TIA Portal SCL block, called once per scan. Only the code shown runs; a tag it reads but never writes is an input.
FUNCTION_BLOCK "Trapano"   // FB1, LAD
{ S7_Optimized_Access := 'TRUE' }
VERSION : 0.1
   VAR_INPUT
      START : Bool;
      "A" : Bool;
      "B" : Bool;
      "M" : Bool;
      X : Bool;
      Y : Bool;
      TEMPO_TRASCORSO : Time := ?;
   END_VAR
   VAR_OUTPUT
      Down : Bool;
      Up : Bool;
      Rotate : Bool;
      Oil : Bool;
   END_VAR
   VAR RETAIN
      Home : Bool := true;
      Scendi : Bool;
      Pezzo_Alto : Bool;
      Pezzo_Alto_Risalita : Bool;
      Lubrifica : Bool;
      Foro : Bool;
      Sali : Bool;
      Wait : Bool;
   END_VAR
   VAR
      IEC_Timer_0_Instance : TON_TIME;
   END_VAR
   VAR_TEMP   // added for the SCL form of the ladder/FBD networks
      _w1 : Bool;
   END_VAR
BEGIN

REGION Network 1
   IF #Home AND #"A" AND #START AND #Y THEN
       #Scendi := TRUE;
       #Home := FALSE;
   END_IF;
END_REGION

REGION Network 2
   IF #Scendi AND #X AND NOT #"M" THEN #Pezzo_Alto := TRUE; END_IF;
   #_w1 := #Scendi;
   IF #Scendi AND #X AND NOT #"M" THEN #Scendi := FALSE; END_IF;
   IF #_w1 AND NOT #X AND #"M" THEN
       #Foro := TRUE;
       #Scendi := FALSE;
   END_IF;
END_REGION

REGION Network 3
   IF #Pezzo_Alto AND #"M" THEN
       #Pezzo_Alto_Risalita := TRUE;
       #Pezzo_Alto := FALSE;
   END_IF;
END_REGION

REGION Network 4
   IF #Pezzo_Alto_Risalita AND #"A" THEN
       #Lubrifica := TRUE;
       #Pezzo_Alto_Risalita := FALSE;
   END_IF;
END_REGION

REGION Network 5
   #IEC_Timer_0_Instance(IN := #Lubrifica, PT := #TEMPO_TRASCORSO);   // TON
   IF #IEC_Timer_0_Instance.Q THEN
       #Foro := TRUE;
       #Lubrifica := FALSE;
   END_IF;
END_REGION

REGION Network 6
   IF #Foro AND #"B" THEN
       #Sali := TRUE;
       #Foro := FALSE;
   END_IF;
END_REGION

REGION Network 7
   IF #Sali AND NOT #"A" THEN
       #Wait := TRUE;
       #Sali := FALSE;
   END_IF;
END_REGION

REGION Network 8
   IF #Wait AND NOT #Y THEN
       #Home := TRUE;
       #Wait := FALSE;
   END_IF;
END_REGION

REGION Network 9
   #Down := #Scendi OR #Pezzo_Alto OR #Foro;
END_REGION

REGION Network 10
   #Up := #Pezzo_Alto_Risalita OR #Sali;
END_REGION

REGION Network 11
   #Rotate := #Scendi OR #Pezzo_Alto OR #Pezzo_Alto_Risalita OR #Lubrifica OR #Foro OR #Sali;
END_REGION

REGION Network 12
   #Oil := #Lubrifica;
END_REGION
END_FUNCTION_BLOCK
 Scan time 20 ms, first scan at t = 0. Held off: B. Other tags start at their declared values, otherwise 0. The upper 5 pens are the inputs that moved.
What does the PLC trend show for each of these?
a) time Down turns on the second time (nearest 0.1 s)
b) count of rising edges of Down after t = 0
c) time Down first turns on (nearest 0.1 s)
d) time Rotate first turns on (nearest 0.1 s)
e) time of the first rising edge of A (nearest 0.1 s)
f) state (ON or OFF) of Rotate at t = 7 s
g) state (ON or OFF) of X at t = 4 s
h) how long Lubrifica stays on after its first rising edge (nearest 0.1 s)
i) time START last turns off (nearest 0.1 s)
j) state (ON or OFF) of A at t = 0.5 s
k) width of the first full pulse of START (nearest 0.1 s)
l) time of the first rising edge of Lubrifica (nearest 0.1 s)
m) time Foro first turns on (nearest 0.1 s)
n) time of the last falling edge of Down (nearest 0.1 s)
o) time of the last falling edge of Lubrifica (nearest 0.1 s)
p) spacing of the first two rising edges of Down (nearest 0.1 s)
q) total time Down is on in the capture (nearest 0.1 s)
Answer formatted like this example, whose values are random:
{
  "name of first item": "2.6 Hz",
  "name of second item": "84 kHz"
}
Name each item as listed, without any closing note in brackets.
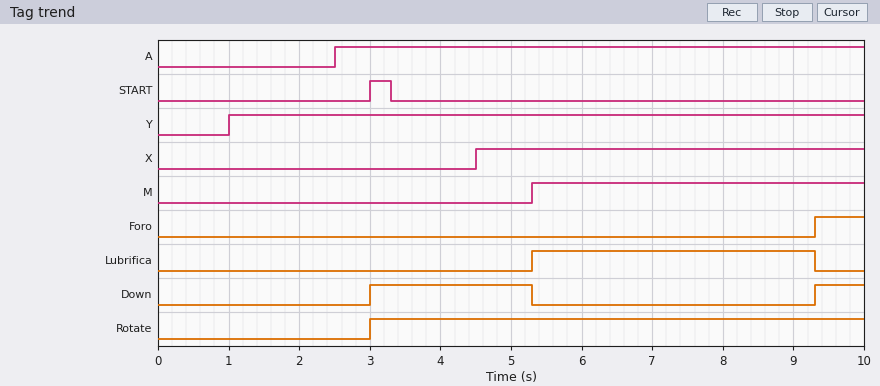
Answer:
{
  "time Down turns on the second time": "9.3 s",
  "count of rising edges of Down after t = 0": "2",
  "time Down first turns on": "3.0 s",
  "time Rotate first turns on": "3.0 s",
  "time of the first rising edge of A": "2.5 s",
  "state (ON or OFF) of Rotate at t = 7 s": "ON",
  "state (ON or OFF) of X at t = 4 s": "OFF",
  "how long Lubrifica stays on after its first rising edge": "4.0 s",
  "time START last turns off": "3.3 s",
  "state (ON or OFF) of A at t = 0.5 s": "OFF",
  "width of the first full pulse of START": "0.3 s",
  "time of the first rising edge of Lubrifica": "5.3 s",
  "time Foro first turns on": "9.3 s",
  "time of the last falling edge of Down": "5.3 s",
  "time of the last falling edge of Lubrifica": "9.3 s",
  "spacing of the first two rising edges of Down": "6.3 s",
  "total time Down is on in the capture": "3.0 s"
}
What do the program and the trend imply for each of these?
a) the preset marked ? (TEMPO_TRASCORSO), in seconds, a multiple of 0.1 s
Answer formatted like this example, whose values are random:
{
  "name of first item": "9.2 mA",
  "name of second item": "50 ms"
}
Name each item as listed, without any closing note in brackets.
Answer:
{
  "the preset marked ? (TEMPO_TRASCORSO), in seconds, a multiple of 0.1 s": "4.0 s"
}
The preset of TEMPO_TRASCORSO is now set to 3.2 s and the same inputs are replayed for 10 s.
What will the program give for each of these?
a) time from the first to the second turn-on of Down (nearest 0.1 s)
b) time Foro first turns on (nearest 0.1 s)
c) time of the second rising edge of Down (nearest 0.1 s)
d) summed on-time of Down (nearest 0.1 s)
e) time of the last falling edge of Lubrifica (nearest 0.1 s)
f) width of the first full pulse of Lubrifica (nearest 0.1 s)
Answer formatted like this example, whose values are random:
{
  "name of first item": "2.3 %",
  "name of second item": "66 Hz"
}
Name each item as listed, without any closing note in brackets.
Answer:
{
  "time from the first to the second turn-on of Down": "5.5 s",
  "time Foro first turns on": "8.5 s",
  "time of the second rising edge of Down": "8.5 s",
  "summed on-time of Down": "3.8 s",
  "time of the last falling edge of Lubrifica": "8.5 s",
  "width of the first full pulse of Lubrifica": "3.2 s"
}
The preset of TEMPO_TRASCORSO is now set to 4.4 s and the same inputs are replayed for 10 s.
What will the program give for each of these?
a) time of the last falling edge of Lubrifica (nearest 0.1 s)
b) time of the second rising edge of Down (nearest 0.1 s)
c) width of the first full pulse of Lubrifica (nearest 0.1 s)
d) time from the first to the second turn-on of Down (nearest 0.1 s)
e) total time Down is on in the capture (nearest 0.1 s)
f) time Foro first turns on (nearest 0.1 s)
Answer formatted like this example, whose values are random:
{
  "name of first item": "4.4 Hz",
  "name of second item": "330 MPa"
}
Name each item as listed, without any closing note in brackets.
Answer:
{
  "time of the last falling edge of Lubrifica": "9.7 s",
  "time of the second rising edge of Down": "9.7 s",
  "width of the first full pulse of Lubrifica": "4.4 s",
  "time from the first to the second turn-on of Down": "6.7 s",
  "total time Down is on in the capture": "2.6 s",
  "time Foro first turns on": "9.7 s"
}
